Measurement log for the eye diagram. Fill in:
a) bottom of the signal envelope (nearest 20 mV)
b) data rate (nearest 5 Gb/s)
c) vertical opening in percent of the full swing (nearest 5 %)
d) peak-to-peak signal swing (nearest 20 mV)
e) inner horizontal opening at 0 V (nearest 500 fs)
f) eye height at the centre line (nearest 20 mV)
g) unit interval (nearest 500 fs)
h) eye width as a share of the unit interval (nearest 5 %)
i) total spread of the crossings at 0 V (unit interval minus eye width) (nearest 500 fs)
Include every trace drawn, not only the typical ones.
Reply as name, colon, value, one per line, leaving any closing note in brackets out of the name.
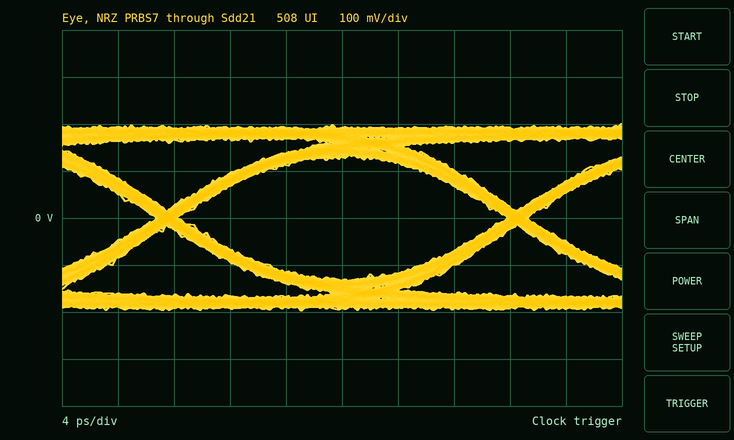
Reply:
bottom of the signal envelope: -200 mV
data rate: 40 Gb/s
vertical opening in percent of the full swing: 65 %
peak-to-peak signal swing: 400 mV
inner horizontal opening at 0 V: 23.5 ps
eye height at the centre line: 260 mV
unit interval: 25.0 ps
eye width as a share of the unit interval: 95 %
total spread of the crossings at 0 V (unit interval minus eye width): 1.5 ps
